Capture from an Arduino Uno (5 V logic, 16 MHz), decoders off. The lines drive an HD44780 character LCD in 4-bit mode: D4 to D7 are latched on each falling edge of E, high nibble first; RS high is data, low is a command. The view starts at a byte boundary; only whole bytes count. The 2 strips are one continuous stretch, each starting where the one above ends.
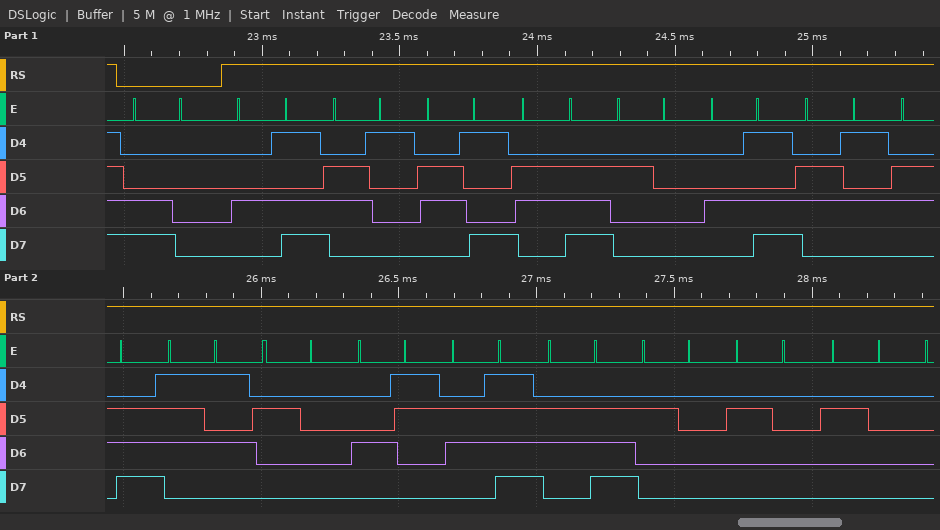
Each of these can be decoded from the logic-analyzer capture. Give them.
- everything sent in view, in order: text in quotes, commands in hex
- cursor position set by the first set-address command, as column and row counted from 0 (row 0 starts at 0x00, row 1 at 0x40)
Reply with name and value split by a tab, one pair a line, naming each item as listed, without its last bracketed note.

everything sent in view, in order: text in quotes, commands in hex	0xC0 "Main Menu Con   "
cursor position set by the first set-address command, as column and row counted from 0	column 0, row 1
